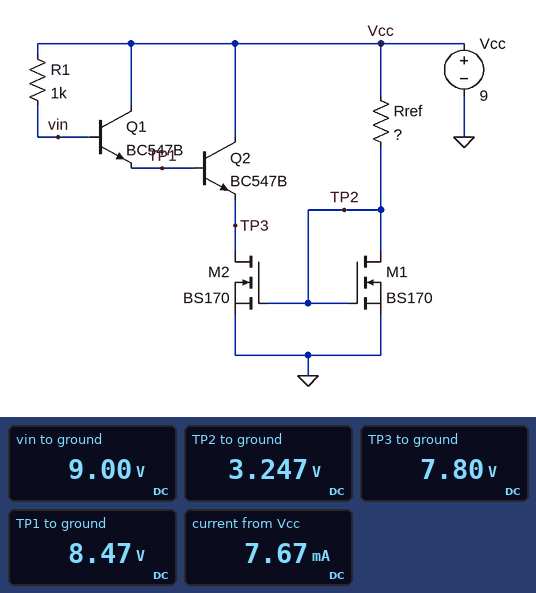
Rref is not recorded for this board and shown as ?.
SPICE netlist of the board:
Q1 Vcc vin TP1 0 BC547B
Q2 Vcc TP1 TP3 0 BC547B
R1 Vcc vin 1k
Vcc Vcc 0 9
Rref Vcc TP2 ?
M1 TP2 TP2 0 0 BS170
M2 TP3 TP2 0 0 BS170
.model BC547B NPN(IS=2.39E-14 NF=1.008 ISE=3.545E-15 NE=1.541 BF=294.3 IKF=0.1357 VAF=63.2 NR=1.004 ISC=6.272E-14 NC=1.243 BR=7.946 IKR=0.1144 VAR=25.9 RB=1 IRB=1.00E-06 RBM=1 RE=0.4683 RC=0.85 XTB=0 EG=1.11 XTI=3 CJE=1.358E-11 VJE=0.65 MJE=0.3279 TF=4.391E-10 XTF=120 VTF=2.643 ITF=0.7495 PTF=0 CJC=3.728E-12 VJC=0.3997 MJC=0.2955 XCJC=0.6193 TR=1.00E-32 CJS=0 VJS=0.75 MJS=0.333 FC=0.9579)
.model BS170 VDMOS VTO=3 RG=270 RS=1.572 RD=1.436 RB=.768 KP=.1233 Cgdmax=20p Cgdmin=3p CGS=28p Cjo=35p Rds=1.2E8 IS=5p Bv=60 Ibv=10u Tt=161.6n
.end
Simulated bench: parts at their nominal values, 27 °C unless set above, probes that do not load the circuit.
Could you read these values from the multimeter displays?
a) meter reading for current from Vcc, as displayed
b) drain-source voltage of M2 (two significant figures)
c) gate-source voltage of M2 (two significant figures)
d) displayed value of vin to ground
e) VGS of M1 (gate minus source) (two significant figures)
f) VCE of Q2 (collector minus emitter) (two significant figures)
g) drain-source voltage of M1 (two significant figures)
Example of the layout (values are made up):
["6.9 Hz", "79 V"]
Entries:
["7.67 mA", "7.8 V", "3.2 V", "9.00 V", "3.2 V", "1.2 V", "3.2 V"]
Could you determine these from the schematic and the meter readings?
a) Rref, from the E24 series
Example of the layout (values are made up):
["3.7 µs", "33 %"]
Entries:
["1.5 kΩ"]
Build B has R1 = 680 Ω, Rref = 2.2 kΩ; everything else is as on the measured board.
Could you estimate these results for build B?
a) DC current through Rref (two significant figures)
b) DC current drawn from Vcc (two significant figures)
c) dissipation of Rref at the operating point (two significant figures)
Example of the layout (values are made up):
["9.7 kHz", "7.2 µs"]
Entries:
["2.6 mA", "5.3 mA", "15 mW"]
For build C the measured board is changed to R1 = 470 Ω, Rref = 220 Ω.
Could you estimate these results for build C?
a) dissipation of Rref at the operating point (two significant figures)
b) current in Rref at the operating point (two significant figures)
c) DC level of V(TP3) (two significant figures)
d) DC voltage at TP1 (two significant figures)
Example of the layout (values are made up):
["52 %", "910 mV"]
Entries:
["130 mW", "24 mA", "7.7 V", "8.4 V"]
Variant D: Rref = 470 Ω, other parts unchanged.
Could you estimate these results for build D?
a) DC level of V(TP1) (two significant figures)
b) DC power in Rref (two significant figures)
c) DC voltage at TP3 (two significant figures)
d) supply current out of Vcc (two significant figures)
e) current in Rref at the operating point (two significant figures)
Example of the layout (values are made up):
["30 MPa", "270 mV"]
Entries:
["8.4 V", "65 mW", "7.7 V", "24 mA", "12 mA"]
